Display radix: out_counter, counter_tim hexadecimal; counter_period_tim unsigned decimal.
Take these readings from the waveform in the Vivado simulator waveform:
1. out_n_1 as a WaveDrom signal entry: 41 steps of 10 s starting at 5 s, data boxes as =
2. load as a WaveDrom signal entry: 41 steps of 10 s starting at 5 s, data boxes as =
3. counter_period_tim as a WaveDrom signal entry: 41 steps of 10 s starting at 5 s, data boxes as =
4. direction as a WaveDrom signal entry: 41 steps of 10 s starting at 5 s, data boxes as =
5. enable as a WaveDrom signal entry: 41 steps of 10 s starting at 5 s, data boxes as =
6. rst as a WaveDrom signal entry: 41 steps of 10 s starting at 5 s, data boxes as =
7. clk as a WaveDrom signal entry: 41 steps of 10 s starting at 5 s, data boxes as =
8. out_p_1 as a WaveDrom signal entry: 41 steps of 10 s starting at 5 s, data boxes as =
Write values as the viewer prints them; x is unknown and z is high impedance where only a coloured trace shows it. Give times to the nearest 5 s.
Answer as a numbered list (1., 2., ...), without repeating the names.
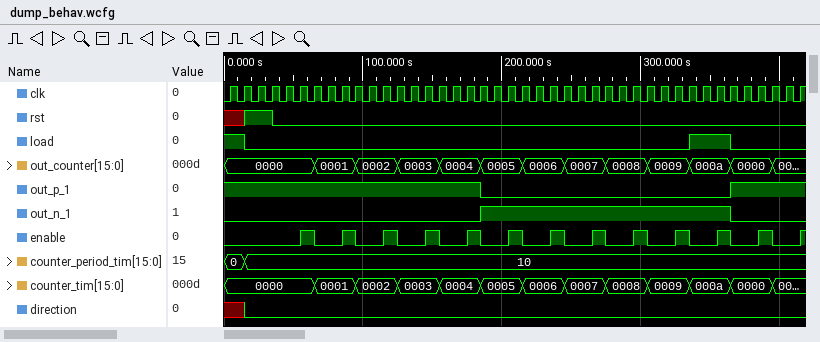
1. {name: 'out_n_1', wave: '0.................1.................0....'}
2. {name: 'load', wave: '10...............................1..0....'}
3. {name: 'counter_period_tim', wave: '==.......................................', data: '0 10'}
4. {name: 'direction', wave: 'x0.......................................'}
5. {name: 'enable', wave: '0....10.10.10.10.10.10.10.10.10.10.10.10.'}
6. {name: 'rst', wave: 'x1.0.....................................'}
7. {name: 'clk', wave: 'p........................................'}
8. {name: 'out_p_1', wave: '1.................0.................1....'}
